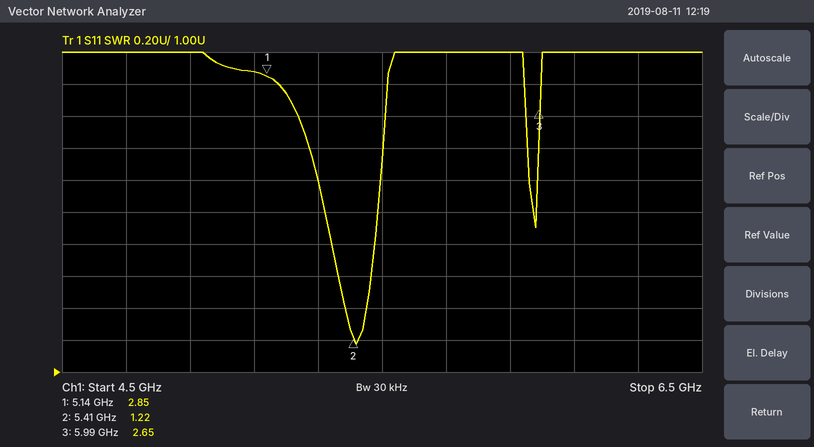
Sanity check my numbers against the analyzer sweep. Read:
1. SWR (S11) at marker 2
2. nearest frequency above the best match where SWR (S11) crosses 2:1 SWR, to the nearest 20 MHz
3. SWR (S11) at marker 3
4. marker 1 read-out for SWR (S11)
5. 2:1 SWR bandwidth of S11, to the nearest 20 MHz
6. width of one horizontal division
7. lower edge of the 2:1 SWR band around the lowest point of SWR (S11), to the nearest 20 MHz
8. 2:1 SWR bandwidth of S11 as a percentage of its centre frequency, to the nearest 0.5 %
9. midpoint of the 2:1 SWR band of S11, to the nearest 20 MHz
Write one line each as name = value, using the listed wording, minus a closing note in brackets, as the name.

SWR (S11) at marker 2 = 1.22
nearest frequency above the best match where SWR (S11) crosses 2:1 SWR, to the nearest 20 MHz = 5.48 GHz
SWR (S11) at marker 3 = 2.65
marker 1 read-out for SWR = 2.85
2:1 SWR bandwidth of S11, to the nearest 20 MHz = 160 MHz
width of one horizontal division = 200 MHz
lower edge of the 2:1 SWR band around the lowest point of SWR (S11), to the nearest 20 MHz = 5.32 GHz
2:1 SWR bandwidth of S11 as a percentage of its centre frequency, to the nearest 0.5 % = 3.0 %
midpoint of the 2:1 SWR band of S11, to the nearest 20 MHz = 5.40 GHz
